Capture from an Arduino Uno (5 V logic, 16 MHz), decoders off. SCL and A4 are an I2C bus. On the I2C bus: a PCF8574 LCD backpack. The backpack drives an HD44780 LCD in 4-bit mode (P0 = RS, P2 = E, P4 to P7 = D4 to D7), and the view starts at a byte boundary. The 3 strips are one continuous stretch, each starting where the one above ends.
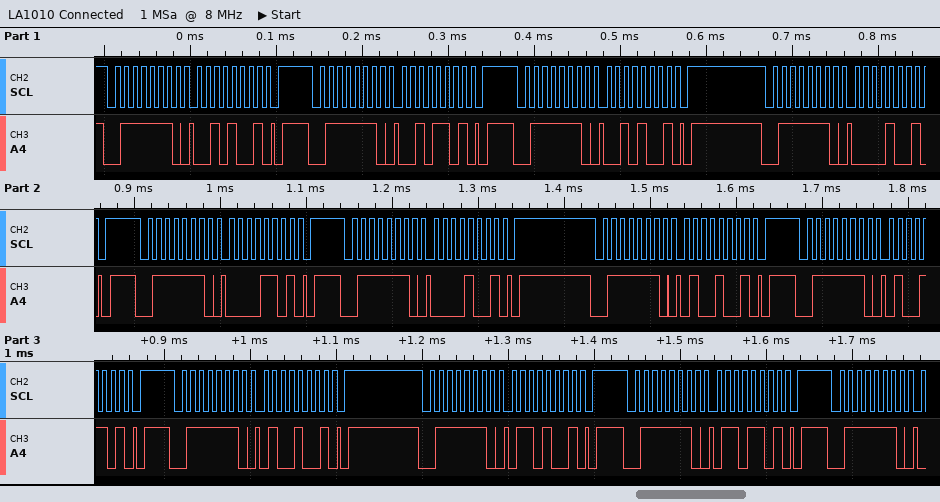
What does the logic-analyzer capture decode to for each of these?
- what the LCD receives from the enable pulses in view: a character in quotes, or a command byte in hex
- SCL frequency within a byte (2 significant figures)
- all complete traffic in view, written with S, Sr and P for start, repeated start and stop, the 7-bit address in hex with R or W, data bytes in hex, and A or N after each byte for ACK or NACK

' '
100 kHz
S 3FW A 29 A P S 3FW A 2D A P S 3FW A 29 A P S 3FW A 09 A P S 3FW A 0D A P S 3FW A 09 A P S 3FW A 49 A P S 3FW A 4D A P S 3FW A 49 A P S 3FW A 69 A P S 3FW A 6D A P S 3FW A
